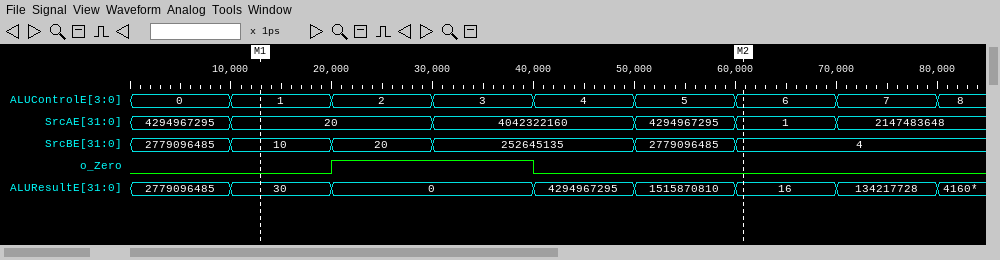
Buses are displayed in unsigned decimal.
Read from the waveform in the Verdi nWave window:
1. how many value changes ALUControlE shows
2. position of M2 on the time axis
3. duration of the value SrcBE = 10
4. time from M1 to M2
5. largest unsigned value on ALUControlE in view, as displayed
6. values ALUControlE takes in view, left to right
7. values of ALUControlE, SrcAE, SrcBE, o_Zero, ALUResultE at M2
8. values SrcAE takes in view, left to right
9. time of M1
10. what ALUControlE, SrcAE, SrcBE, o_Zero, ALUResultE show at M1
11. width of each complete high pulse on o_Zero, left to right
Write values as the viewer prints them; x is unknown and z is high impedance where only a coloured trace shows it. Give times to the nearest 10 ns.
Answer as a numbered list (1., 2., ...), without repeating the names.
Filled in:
1. 8
2. 60 ns
3. 10 ns
4. 50 ns
5. 8
6. 0, 1, 2, 3, 4, 5, 6, 7, 8
7. ALUControlE=6, SrcAE=1, SrcBE=4, o_Zero=0, ALUResultE=16
8. 4294967295, 20, 4042322160, 4294967295, 1, 2147483648
9. 10 ns
10. ALUControlE=1, SrcAE=20, SrcBE=10, o_Zero=0, ALUResultE=30
11. 20 ns
